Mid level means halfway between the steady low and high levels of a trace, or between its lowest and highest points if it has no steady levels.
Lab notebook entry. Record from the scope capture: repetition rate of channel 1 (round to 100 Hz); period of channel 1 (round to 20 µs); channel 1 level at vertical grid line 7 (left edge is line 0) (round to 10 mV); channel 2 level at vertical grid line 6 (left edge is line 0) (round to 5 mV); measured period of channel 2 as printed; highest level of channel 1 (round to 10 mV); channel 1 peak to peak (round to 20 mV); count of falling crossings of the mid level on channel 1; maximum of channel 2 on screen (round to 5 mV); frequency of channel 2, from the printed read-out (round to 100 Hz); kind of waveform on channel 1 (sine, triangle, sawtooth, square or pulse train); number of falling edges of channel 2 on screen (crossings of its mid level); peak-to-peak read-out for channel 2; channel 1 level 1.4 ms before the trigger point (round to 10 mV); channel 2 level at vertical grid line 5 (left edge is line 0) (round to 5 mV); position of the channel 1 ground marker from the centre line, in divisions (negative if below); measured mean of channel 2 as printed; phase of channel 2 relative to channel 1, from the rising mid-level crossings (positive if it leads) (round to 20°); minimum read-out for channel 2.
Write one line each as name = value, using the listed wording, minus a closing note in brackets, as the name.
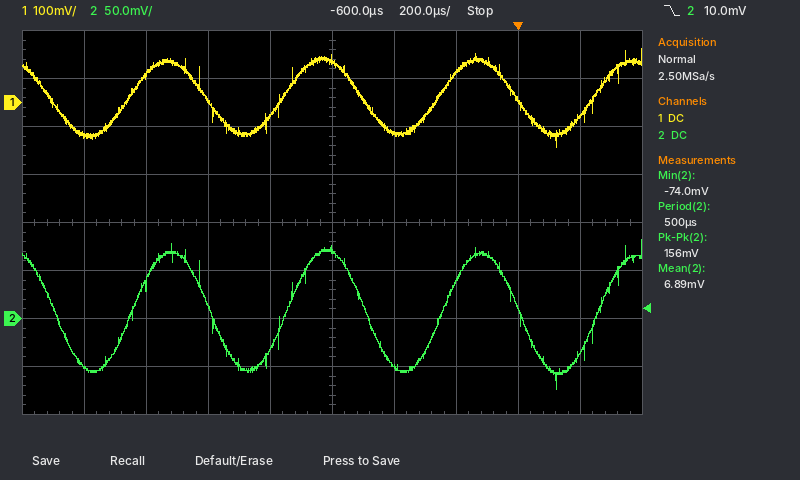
repetition rate of channel 1 = 2.0 kHz
period of channel 1 = 500 µs
channel 1 level at vertical grid line 7 (left edge is line 0) = 60 mV
channel 2 level at vertical grid line 6 (left edge is line 0) = -50 mV
measured period of channel 2 as printed = 500 µs
highest level of channel 1 = 110 mV
channel 1 peak to peak = 200 mV
count of falling crossings of the mid level on channel 1 = 4
maximum of channel 2 on screen = 80 mV
frequency of channel 2, from the printed read-out = 2.0 kHz
kind of waveform on channel 1 = sine
number of falling edges of channel 2 on screen = 4
peak-to-peak read-out for channel 2 = 156 mV
channel 1 level 1.4 ms before the trigger point = -70 mV
channel 2 level at vertical grid line 5 (left edge is line 0) = 70 mV
position of the channel 1 ground marker from the centre line, in divisions = +2.5 div
measured mean of channel 2 as printed = 6.89 mV
phase of channel 2 relative to channel 1, from the rising mid-level crossings (positive if it leads) = 0°
minimum read-out for channel 2 = -74.0 mV
